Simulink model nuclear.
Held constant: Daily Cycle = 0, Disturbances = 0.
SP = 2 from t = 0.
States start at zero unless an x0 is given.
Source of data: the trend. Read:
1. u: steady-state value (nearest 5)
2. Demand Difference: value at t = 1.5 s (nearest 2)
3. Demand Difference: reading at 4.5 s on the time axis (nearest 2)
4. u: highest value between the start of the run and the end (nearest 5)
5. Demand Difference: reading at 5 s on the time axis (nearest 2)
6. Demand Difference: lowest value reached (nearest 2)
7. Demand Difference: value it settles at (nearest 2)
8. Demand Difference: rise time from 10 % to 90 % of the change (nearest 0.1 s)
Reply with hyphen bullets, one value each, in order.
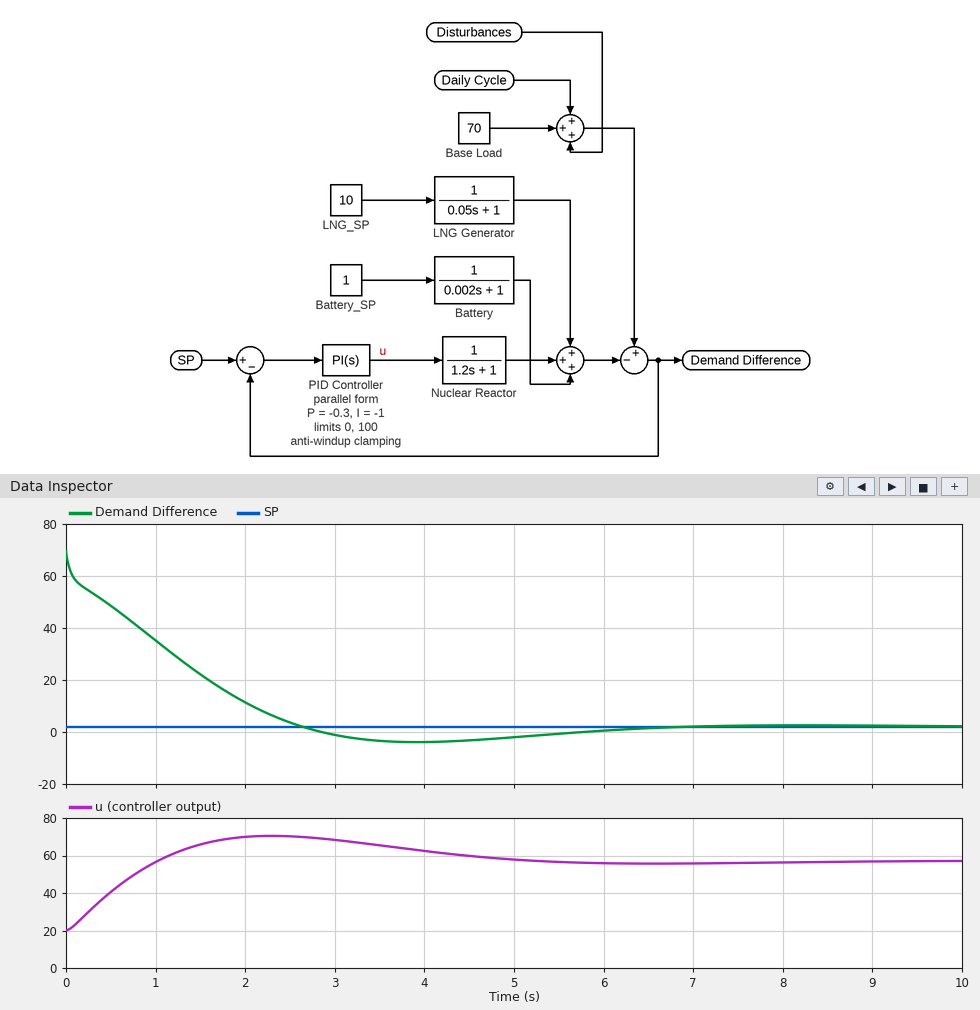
- 55
- 22
- -4
- 70
- -2
- -4
- 2
- 2.1 s
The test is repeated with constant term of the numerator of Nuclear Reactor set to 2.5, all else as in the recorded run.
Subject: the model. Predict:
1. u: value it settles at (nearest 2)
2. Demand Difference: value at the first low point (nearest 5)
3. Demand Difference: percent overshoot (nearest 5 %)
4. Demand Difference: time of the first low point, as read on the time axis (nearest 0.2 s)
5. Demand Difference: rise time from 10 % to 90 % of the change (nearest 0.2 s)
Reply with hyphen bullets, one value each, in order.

- 22
- -10
- 15 %
- 2.2 s
- 1.0 s
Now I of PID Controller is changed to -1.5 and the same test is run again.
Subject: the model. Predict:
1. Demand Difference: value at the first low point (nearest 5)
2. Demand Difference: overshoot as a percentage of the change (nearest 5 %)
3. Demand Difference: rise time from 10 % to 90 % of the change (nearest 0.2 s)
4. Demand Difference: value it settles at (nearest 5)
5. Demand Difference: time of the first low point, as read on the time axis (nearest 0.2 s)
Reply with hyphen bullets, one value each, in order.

- -10
- 15 %
- 1.6 s
- 0
- 3.0 s
